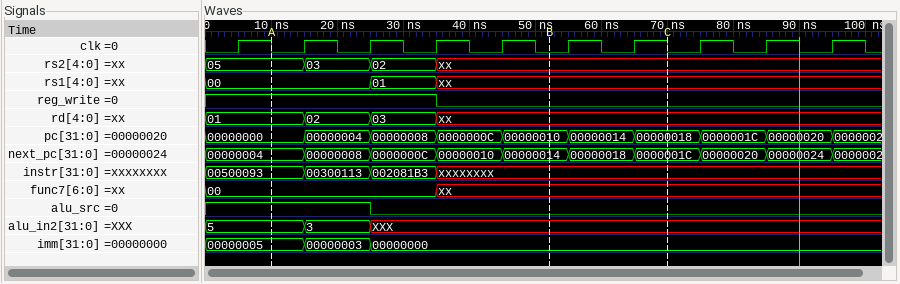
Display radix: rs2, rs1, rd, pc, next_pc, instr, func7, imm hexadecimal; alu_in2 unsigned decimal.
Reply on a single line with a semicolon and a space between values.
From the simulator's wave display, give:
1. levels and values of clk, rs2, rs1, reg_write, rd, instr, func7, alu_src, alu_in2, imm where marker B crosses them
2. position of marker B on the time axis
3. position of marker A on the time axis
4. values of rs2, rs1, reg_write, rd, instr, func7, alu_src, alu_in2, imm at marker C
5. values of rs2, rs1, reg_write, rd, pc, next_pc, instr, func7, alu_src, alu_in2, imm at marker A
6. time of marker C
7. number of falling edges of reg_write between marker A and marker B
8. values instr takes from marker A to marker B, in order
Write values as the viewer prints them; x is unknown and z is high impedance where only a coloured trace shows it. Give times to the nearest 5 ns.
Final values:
clk=0, rs2=xx, rs1=xx, reg_write=0, rd=xx, instr=xxxxxxxx, func7=xx, alu_src=0, alu_in2=XXX, imm=00000000; 50 ns; 10 ns; rs2=xx, rs1=xx, reg_write=0, rd=xx, instr=xxxxxxxx, func7=xx, alu_src=0, alu_in2=XXX, imm=00000000; rs2=05, rs1=00, reg_write=1, rd=01, pc=00000000, next_pc=00000004, instr=00500093, func7=00, alu_src=1, alu_in2=5, imm=00000005; 70 ns; 1; 00500093, 00300113, 002081B3, xxxxxxxx
